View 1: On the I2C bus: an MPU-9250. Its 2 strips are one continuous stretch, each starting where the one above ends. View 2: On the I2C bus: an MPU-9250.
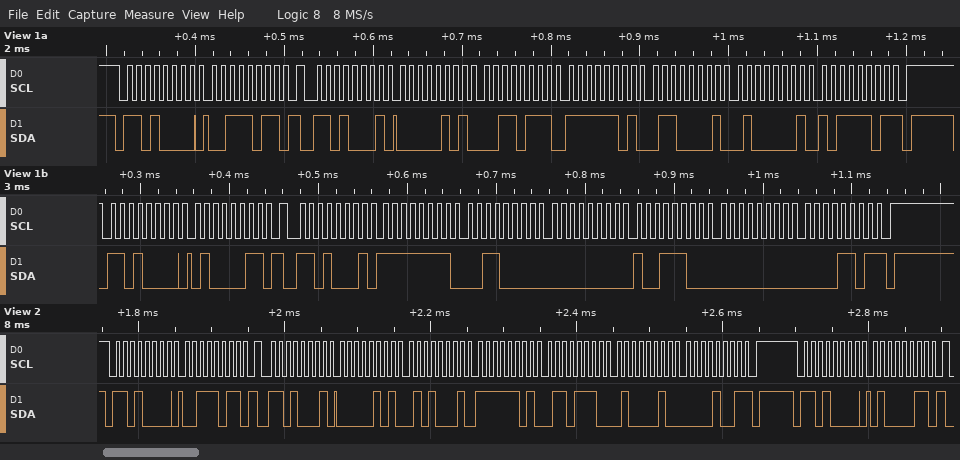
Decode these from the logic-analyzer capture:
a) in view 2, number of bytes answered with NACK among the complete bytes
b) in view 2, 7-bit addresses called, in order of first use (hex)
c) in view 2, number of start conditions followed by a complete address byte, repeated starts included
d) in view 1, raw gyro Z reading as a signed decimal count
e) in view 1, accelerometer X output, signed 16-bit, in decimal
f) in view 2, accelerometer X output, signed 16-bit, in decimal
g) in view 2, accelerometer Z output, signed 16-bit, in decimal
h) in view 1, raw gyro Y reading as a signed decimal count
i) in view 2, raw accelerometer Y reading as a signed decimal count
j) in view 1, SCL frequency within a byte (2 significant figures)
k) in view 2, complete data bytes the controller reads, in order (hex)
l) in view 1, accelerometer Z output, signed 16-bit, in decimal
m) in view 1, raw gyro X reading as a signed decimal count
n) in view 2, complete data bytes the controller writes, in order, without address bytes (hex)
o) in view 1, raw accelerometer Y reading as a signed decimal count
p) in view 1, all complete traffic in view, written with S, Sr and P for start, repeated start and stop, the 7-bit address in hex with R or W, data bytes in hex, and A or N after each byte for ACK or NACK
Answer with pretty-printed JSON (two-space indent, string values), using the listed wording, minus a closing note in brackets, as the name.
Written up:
{
  "in view 2, number of bytes answered with NACK among the complete bytes": "1",
  "in view 2, 7-bit addresses called, in order of first use": "0x68",
  "in view 2, number of start conditions followed by a complete address byte, repeated starts included": "3",
  "in view 1, raw gyro Z reading as a signed decimal count": "13",
  "in view 1, accelerometer X output, signed 16-bit, in decimal": "1335",
  "in view 2, accelerometer X output, signed 16-bit, in decimal": "1361",
  "in view 2, accelerometer Z output, signed 16-bit, in decimal": "16905",
  "in view 1, raw gyro Y reading as a signed decimal count": "156",
  "in view 2, raw accelerometer Y reading as a signed decimal count": "-658",
  "in view 1, SCL frequency within a byte": "100 kHz",
  "in view 2, complete data bytes the controller reads, in order": "05 51 FD 6E 42 09",
  "in view 1, accelerometer Z output, signed 16-bit, in decimal": "16829",
  "in view 1, raw gyro X reading as a signed decimal count": "-208",
  "in view 2, complete data bytes the controller writes, in order, without address bytes": "3B 43",
  "in view 1, raw accelerometer Y reading as a signed decimal count": "-671",
  "in view 1, all complete traffic in view, written with S, Sr and P for start, repeated start and stop, the 7-bit address in hex with R or W, data bytes in hex, and A or N after each byte for ACK or NACK": "S 68W A 3B A Sr 68R A 05 A 37 A FD A 61 A 41 A BD N P S 68W A 43 A Sr 68R A FF A 30 A 00 A 9C A 00 A 0D N P"
}
